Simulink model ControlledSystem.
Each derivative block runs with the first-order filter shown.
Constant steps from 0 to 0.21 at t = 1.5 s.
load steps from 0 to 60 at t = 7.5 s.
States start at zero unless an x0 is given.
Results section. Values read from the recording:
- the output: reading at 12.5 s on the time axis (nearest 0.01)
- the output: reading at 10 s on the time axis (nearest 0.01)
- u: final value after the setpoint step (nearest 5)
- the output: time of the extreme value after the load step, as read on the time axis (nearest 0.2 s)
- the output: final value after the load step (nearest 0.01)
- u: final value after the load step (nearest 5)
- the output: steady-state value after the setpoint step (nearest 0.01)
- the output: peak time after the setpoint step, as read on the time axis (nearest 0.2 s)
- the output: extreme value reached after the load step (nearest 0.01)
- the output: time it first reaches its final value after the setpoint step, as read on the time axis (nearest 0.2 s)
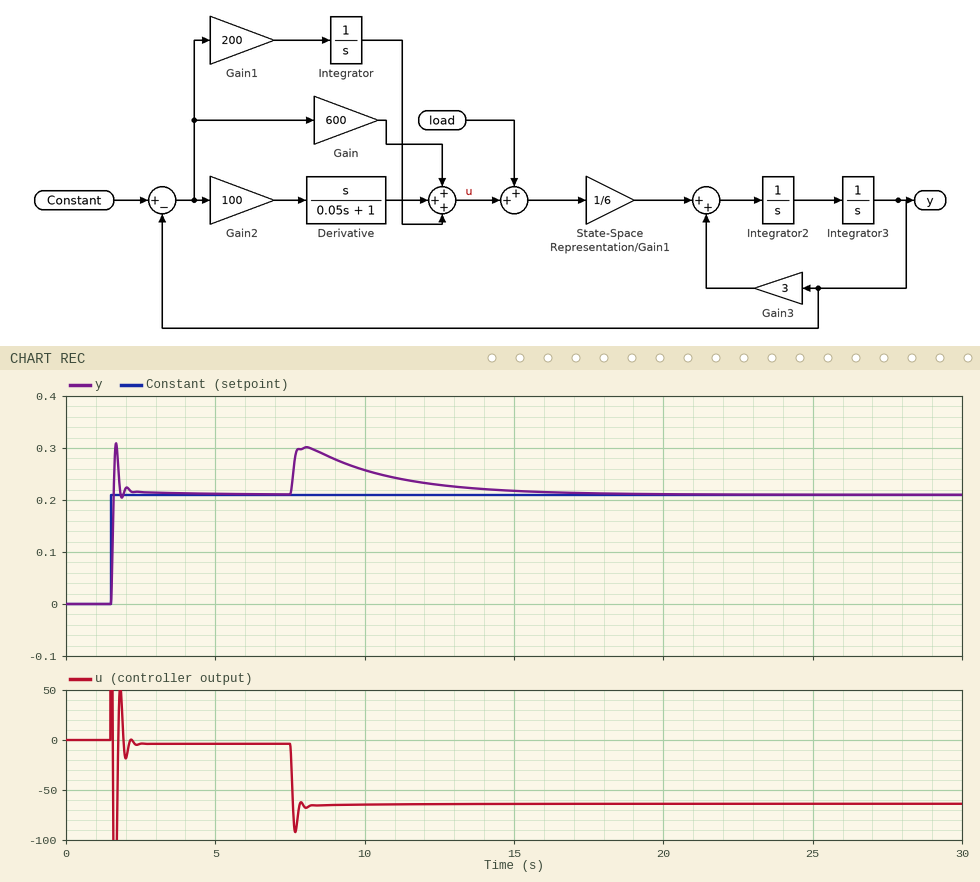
0.23
0.26
-5
8.0 s
0.21
-65
0.21
1.6 s
0.30
1.6 s
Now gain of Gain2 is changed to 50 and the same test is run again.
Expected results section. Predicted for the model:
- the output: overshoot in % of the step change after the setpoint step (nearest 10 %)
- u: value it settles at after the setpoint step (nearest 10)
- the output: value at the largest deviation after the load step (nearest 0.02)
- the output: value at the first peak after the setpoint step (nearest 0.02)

60 %
0
0.34
0.34
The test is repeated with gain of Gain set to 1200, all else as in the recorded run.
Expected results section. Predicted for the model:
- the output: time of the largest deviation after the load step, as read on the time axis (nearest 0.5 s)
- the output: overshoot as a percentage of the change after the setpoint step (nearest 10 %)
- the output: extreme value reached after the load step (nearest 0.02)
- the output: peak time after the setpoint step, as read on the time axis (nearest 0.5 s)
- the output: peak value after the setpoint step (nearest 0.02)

7.5 s
60 %
0.26
1.5 s
0.34
